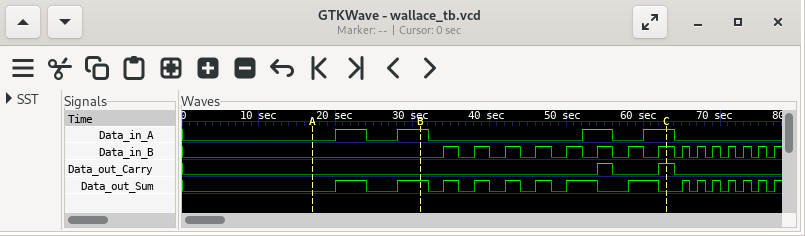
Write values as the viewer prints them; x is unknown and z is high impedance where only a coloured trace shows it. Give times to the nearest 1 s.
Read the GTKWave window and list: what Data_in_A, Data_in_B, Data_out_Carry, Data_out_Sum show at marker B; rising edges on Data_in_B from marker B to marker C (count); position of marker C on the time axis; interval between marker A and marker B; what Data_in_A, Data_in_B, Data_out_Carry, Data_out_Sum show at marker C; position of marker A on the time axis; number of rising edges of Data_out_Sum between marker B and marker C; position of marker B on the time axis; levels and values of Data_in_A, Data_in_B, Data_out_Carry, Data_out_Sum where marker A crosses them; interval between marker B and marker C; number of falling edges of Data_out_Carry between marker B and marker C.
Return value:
Data_in_A=1, Data_in_B=0, Data_out_Carry=0, Data_out_Sum=1
8
63 s
14 s
Data_in_A=1, Data_in_B=1, Data_out_Carry=1, Data_out_Sum=0
17 s
6
31 s
Data_in_A=0, Data_in_B=0, Data_out_Carry=0, Data_out_Sum=0
32 s
1
